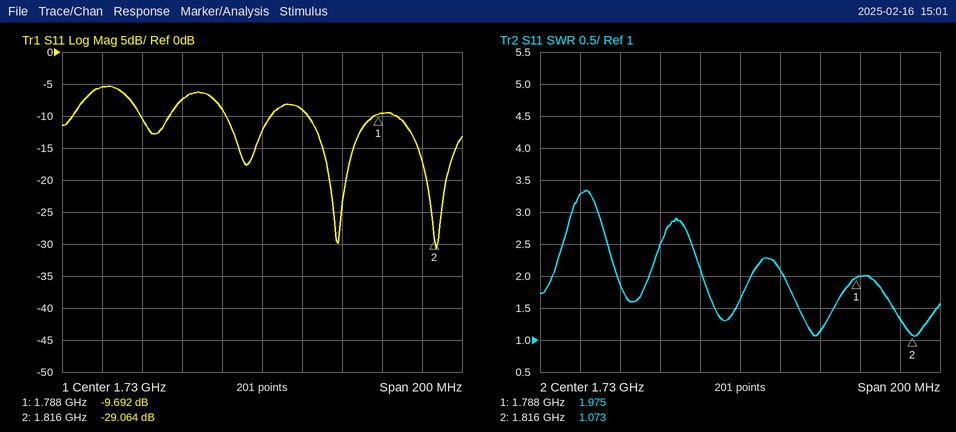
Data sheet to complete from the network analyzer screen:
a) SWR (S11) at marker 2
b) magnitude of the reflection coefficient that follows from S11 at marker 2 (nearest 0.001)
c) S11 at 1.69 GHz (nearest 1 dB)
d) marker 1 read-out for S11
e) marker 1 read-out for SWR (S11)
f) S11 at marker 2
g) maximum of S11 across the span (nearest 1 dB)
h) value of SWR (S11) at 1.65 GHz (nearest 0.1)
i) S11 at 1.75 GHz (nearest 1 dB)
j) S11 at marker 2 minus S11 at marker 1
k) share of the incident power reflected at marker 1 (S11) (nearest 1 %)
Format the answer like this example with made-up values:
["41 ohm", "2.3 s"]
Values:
["1.073", "0.035", "-7 dB", "-9.692 dB", "1.975", "-29.064 dB", "-5 dB", "3.3", "-9 dB", "-19.372 dB", "11 %"]
